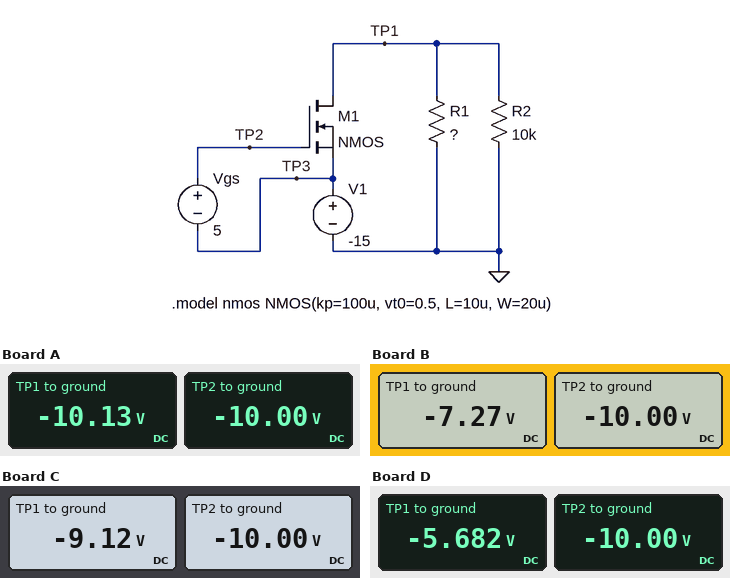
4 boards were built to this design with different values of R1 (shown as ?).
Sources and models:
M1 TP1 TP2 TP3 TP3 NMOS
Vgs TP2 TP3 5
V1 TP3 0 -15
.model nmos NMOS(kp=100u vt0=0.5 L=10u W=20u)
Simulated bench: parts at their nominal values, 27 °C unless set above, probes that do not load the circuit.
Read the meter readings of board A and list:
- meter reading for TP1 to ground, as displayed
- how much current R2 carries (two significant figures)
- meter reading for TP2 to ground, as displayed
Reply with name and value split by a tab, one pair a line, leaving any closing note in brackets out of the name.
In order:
meter reading for TP1 to ground, as displayed	-10.13 V
how much current R2 carries	1.0 mA
meter reading for TP2 to ground, as displayed	-10.00 V
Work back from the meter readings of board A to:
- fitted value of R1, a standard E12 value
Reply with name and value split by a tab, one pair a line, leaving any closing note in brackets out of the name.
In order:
fitted value of R1, a standard E12 value	10 kΩ
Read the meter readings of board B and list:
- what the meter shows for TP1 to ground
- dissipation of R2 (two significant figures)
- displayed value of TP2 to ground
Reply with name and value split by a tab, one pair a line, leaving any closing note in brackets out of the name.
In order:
what the meter shows for TP1 to ground	-7.27 V
dissipation of R2	5.3 mW
displayed value of TP2 to ground	-10.00 V
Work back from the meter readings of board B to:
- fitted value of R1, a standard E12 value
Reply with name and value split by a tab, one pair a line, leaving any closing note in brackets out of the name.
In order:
fitted value of R1, a standard E12 value	5.6 kΩ
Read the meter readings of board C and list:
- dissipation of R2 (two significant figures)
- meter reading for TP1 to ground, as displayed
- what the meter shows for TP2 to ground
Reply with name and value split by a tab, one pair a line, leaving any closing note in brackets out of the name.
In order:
dissipation of R2	8.3 mW
meter reading for TP1 to ground, as displayed	-9.12 V
what the meter shows for TP2 to ground	-10.00 V
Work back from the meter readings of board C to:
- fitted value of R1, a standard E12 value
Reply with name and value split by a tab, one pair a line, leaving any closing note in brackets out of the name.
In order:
fitted value of R1, a standard E12 value	8.2 kΩ
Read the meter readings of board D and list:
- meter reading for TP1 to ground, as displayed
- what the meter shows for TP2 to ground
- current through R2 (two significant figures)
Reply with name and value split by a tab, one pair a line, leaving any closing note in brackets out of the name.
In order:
meter reading for TP1 to ground, as displayed	-5.682 V
what the meter shows for TP2 to ground	-10.00 V
current through R2	570 µA
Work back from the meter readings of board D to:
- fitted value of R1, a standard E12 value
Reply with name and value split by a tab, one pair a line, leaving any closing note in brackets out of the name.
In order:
fitted value of R1, a standard E12 value	3.9 kΩ
